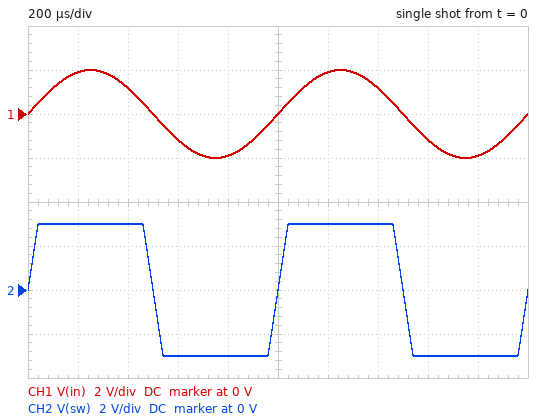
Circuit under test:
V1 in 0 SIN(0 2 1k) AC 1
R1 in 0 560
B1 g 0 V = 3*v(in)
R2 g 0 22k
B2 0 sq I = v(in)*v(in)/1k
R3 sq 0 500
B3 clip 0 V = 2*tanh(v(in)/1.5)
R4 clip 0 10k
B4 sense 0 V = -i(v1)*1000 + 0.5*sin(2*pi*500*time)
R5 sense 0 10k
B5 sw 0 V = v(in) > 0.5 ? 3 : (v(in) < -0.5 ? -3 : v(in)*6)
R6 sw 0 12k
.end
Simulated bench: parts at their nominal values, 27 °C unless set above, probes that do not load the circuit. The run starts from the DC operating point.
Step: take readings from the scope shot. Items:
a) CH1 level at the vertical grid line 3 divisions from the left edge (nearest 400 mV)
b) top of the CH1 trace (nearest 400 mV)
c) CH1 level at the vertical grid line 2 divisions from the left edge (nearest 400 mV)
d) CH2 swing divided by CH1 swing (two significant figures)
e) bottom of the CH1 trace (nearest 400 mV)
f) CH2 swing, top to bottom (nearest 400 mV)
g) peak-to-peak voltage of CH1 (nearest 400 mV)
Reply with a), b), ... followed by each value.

a) -1.2 V
b) 2.0 V
c) 1.2 V
d) 1.5
e) -2.0 V
f) 6.0 V
g) 4.0 V
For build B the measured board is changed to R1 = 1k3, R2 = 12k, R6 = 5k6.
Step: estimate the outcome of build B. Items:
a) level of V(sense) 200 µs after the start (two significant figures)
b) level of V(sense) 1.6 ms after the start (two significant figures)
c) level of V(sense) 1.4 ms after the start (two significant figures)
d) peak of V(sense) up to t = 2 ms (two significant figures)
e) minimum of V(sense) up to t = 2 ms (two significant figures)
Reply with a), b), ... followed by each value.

a) 1.8 V
b) -1.4 V
c) 430 mV
d) 1.9 V
e) -1.9 V
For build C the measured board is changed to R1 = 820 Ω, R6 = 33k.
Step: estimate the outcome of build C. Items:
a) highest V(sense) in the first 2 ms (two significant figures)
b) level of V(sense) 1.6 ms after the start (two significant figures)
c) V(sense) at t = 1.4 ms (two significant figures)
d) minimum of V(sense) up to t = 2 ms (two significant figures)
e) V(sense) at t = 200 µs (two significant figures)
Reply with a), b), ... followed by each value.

a) 2.8 V
b) -1.9 V
c) 960 mV
d) -2.8 V
e) 2.6 V
